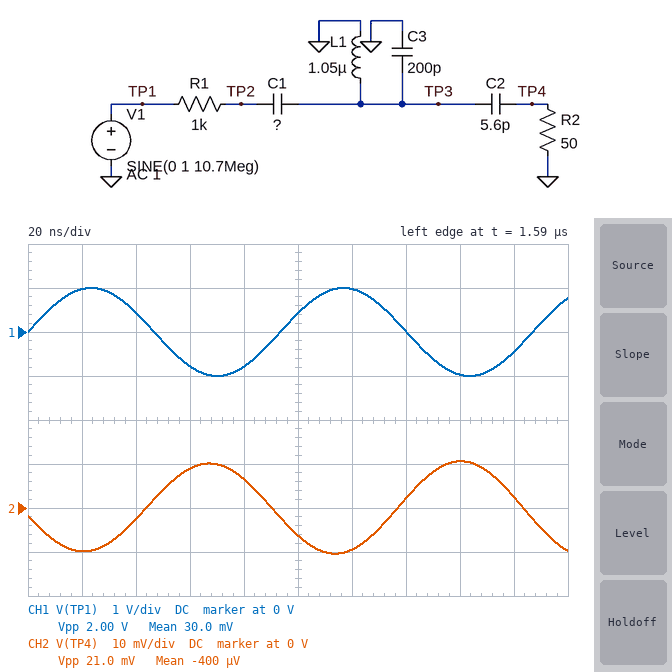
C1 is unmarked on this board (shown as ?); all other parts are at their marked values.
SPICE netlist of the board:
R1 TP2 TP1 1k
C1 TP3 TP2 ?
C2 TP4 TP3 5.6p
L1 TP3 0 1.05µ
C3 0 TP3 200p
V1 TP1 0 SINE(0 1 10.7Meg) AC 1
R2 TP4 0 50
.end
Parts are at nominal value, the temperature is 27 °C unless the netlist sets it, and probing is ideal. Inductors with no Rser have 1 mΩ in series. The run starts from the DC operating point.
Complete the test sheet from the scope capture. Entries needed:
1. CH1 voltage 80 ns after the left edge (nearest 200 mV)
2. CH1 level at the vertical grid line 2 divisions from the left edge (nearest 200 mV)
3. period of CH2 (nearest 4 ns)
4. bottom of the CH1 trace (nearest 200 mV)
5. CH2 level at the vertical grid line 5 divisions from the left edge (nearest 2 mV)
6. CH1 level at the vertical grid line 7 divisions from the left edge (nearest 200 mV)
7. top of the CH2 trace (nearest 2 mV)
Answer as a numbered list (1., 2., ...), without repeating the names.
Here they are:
1. -800 mV
2. 400 mV
3. 92 ns
4. -1.0 V
5. -6 mV
6. 0 V
7. 10 mV
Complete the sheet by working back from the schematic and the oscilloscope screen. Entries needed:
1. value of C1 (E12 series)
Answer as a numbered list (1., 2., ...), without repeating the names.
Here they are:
1. 2.2 pF
